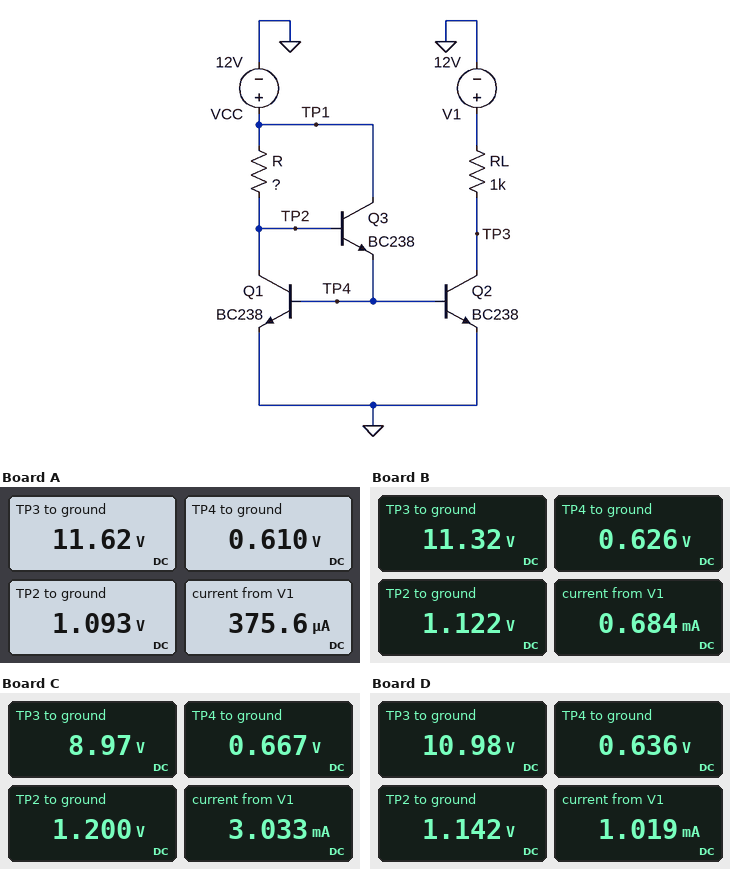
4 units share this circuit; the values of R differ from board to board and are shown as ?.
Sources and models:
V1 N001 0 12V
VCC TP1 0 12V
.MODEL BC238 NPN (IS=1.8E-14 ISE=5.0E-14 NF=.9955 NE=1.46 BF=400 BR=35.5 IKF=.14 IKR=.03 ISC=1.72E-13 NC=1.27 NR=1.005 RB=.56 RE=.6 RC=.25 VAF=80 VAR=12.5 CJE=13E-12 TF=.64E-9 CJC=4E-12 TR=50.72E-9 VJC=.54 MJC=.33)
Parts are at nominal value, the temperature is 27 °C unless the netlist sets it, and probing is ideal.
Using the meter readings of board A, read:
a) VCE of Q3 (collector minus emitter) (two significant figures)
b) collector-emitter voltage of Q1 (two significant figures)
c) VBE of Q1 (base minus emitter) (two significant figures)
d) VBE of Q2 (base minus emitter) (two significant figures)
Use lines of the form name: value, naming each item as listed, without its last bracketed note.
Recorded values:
VCE of Q3 (collector minus emitter): 11 V
collector-emitter voltage of Q1: 1.1 V
VBE of Q1 (base minus emitter): 610 mV
VBE of Q2 (base minus emitter): 610 mV
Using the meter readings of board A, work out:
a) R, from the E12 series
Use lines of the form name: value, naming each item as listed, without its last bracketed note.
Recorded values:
R, from the E12 series: 33 kΩ
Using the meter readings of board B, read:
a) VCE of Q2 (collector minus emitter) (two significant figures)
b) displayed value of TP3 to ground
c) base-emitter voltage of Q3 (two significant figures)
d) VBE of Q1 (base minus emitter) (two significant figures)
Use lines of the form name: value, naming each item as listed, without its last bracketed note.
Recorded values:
VCE of Q2 (collector minus emitter): 11 V
displayed value of TP3 to ground: 11.32 V
base-emitter voltage of Q3: 500 mV
VBE of Q1 (base minus emitter): 630 mV
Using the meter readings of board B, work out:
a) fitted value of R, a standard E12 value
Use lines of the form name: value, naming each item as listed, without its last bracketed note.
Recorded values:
fitted value of R, a standard E12 value: 18 kΩ
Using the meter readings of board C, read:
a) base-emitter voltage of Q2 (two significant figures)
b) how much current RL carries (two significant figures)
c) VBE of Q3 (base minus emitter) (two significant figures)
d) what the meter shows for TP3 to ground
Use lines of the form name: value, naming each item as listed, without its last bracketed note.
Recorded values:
base-emitter voltage of Q2: 670 mV
how much current RL carries: 3.0 mA
VBE of Q3 (base minus emitter): 530 mV
what the meter shows for TP3 to ground: 8.97 V
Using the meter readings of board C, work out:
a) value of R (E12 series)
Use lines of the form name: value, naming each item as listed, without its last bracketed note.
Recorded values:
value of R: 3.9 kΩ
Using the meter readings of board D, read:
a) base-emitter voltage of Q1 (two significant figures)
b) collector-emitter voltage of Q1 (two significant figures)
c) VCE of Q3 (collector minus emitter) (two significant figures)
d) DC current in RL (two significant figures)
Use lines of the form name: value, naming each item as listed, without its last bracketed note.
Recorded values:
base-emitter voltage of Q1: 640 mV
collector-emitter voltage of Q1: 1.1 V
VCE of Q3 (collector minus emitter): 11 V
DC current in RL: 1.0 mA
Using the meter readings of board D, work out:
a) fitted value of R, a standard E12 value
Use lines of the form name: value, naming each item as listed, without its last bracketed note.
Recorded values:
fitted value of R, a standard E12 value: 12 kΩ
